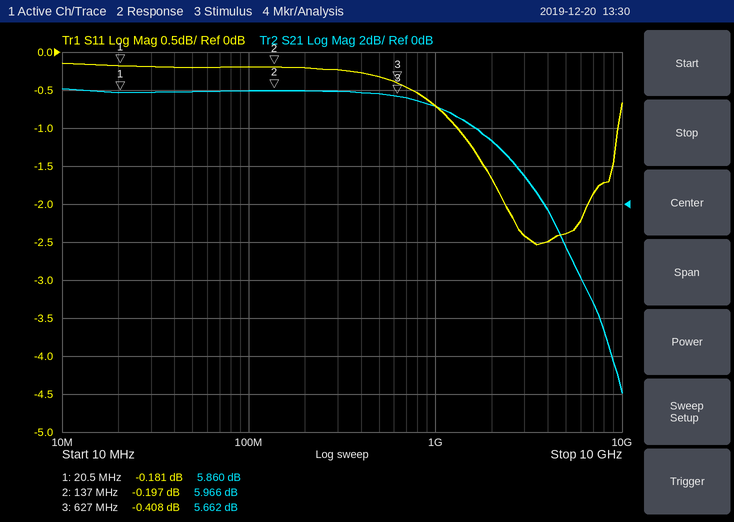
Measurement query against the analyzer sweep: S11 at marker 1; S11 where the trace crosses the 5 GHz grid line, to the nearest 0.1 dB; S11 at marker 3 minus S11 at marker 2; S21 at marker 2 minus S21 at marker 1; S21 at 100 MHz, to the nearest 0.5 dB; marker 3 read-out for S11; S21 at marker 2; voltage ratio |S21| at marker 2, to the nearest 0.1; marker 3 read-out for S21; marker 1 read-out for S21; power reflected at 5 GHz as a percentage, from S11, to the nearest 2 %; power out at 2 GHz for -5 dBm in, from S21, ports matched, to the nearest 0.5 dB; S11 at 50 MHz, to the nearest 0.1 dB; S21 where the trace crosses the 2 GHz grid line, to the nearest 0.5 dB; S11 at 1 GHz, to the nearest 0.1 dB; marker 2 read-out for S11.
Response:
-0.181 dB
-2.4 dB
-0.211 dB
0.106 dB
6.0 dB
-0.408 dB
5.966 dB
2.0
5.662 dB
5.860 dB
58 %
-1.5 dBm
-0.2 dB
3.5 dB
-0.7 dB
-0.197 dB
